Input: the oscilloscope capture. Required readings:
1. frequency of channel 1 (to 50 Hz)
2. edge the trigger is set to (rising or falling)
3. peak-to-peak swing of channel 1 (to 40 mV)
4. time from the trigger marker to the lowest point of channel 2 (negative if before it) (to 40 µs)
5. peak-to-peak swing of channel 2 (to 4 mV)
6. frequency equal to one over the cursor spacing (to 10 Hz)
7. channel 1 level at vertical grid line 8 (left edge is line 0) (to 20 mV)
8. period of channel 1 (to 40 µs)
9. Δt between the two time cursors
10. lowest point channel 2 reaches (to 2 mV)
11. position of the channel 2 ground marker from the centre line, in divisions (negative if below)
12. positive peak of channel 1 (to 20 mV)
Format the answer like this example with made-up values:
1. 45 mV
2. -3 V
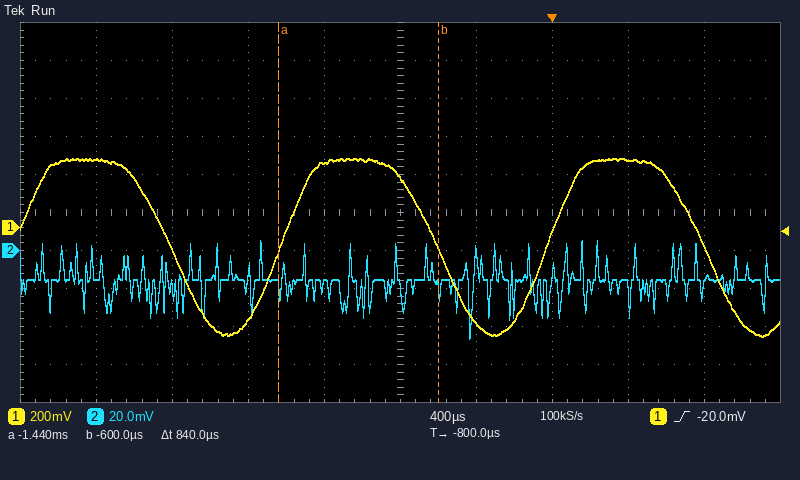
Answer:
1. 700 Hz
2. rising
3. 920 mV
4. -440 µs
5. 52 mV
6. 1.19 kHz
7. 360 mV
8. 1.40 ms
9. 840 µs
10. -46 mV
11. -1.0 div
12. 360 mV
